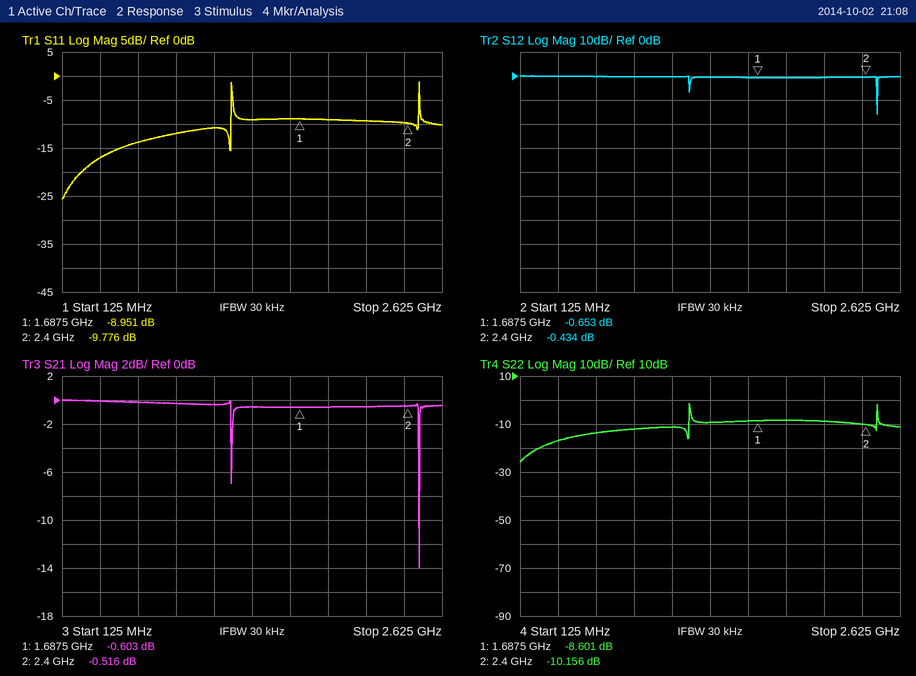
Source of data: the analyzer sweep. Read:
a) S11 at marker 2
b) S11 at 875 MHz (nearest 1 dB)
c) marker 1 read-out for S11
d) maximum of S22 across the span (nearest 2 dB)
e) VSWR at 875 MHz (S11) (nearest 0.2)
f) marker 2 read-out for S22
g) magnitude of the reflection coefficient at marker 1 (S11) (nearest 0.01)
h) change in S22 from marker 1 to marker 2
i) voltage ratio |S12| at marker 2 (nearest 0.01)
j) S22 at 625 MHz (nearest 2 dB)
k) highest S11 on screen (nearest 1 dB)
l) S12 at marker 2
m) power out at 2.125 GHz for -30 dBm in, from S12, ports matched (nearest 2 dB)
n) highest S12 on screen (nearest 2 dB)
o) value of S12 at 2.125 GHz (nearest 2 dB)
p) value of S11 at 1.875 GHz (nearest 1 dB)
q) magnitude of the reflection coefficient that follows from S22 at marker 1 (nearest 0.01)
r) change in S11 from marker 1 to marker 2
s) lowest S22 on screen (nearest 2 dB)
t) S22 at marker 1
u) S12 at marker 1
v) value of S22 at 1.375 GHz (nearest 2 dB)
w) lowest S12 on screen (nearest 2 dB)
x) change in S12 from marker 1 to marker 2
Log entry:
-9.776 dB
-12 dB
-8.951 dB
-2 dB
1.6
-10.156 dB
0.36
-1.555 dB
0.95
-14 dB
-1 dB
-0.434 dB
-30 dBm
0 dB
0 dB
-9 dB
0.37
-0.825 dB
-26 dB
-8.601 dB
-0.653 dB
-10 dB
-16 dB
0.219 dB
